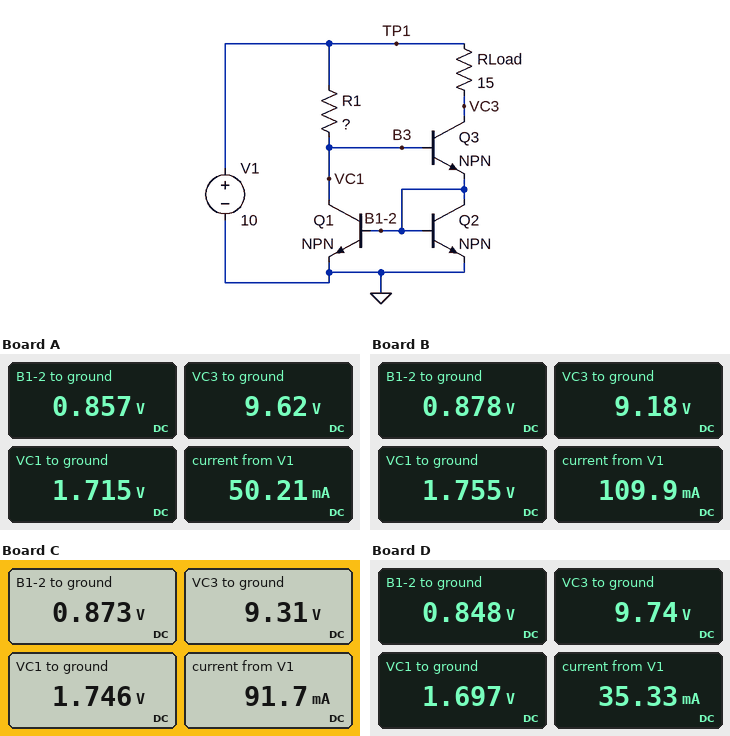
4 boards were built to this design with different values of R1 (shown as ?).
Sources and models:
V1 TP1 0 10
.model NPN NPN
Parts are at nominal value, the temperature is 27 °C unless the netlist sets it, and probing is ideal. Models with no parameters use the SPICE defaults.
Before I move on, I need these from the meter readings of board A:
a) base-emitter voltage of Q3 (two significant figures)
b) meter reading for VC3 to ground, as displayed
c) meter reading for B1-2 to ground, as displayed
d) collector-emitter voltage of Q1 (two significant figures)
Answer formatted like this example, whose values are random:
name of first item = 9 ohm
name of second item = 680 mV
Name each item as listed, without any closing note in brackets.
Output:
base-emitter voltage of Q3 = 860 mV
meter reading for VC3 to ground, as displayed = 9.62 V
meter reading for B1-2 to ground, as displayed = 0.857 V
collector-emitter voltage of Q1 = 1.7 V
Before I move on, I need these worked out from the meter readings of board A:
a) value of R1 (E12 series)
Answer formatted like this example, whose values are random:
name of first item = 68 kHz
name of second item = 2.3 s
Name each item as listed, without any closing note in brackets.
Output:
value of R1 = 330 Ω
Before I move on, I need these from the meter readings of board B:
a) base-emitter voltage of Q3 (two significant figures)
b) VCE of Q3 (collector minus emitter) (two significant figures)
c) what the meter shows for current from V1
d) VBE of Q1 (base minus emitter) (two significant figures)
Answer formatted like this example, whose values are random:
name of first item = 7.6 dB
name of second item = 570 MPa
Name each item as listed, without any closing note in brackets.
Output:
base-emitter voltage of Q3 = 880 mV
VCE of Q3 (collector minus emitter) = 8.3 V
what the meter shows for current from V1 = 109.9 mA
VBE of Q1 (base minus emitter) = 880 mV
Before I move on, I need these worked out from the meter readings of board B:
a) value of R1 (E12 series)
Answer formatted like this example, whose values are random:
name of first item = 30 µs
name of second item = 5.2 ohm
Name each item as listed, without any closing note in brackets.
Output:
value of R1 = 150 Ω
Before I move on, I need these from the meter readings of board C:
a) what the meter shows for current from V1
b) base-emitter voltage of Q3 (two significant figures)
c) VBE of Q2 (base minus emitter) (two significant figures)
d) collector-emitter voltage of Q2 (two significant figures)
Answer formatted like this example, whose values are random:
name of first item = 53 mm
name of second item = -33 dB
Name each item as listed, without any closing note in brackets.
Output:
what the meter shows for current from V1 = 91.7 mA
base-emitter voltage of Q3 = 870 mV
VBE of Q2 (base minus emitter) = 870 mV
collector-emitter voltage of Q2 = 870 mV
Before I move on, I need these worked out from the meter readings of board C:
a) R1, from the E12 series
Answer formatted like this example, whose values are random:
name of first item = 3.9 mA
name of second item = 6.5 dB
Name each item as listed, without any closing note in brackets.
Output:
R1, from the E12 series = 180 Ω
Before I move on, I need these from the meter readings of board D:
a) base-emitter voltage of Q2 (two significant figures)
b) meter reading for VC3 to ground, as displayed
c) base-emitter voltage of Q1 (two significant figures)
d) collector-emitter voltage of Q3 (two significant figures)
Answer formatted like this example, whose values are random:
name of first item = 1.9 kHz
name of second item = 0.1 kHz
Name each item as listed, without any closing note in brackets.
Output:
base-emitter voltage of Q2 = 850 mV
meter reading for VC3 to ground, as displayed = 9.74 V
base-emitter voltage of Q1 = 850 mV
collector-emitter voltage of Q3 = 8.9 V
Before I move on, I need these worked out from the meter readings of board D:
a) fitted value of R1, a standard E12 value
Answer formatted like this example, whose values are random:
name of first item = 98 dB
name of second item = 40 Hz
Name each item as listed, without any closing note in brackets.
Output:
fitted value of R1, a standard E12 value = 470 Ω
